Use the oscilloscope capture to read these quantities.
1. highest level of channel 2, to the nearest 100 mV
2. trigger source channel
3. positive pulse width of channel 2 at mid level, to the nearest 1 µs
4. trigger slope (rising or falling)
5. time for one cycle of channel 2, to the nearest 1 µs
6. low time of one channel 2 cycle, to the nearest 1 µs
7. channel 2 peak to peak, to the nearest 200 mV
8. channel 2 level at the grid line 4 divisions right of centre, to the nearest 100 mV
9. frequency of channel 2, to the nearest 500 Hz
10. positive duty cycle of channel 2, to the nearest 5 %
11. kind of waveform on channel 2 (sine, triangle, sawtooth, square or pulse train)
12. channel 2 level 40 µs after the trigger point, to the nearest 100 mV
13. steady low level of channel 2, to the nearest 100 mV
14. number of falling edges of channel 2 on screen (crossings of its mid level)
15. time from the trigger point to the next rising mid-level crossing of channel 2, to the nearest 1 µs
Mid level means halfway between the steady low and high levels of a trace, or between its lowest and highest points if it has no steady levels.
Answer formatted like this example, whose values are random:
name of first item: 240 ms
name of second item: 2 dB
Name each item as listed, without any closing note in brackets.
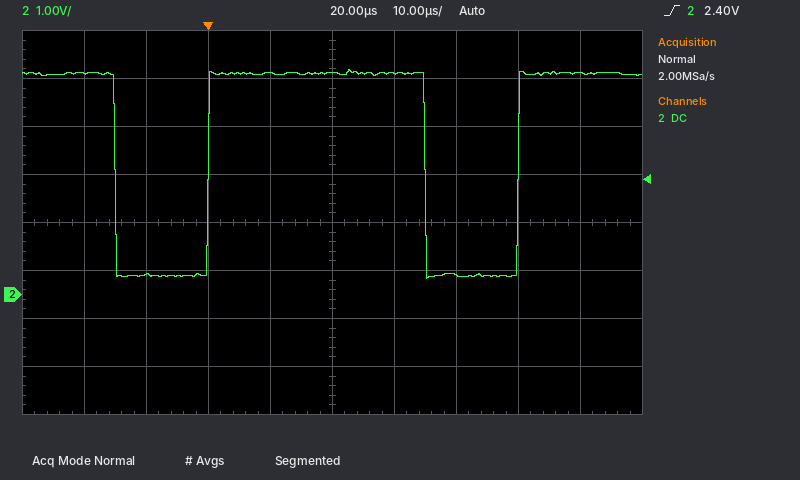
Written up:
highest level of channel 2, to the nearest 100 mV: 4.7 V
trigger source channel: channel 2
positive pulse width of channel 2 at mid level, to the nearest 1 µs: 35 µs
trigger slope: rising
time for one cycle of channel 2, to the nearest 1 µs: 50 µs
low time of one channel 2 cycle, to the nearest 1 µs: 15 µs
channel 2 peak to peak, to the nearest 200 mV: 4.4 V
channel 2 level at the grid line 4 divisions right of centre, to the nearest 100 mV: 4.6 V
frequency of channel 2, to the nearest 500 Hz: 20.0 kHz
positive duty cycle of channel 2, to the nearest 5 %: 70 %
kind of waveform on channel 2: pulse train
channel 2 level 40 µs after the trigger point, to the nearest 100 mV: 400 mV
steady low level of channel 2, to the nearest 100 mV: 400 mV
number of falling edges of channel 2 on screen: 2
time from the trigger point to the next rising mid-level crossing of channel 2, to the nearest 1 µs: 50 µs
